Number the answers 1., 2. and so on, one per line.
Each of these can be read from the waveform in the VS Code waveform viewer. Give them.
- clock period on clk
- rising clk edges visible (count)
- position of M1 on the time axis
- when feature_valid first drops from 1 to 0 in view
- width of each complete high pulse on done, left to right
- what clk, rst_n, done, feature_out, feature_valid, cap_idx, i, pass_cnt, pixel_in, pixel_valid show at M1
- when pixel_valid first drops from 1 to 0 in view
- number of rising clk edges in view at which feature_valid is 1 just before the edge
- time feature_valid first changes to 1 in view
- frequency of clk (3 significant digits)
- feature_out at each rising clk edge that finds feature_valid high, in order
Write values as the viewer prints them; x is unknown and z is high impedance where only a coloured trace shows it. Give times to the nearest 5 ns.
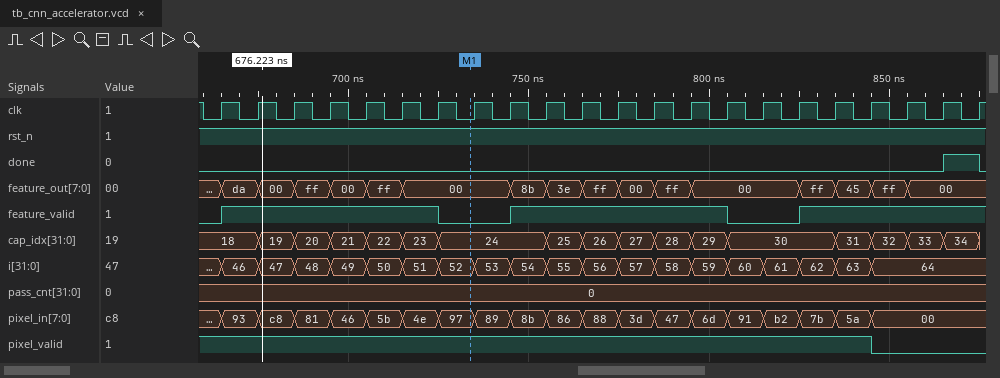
1. 10 ns
2. 22
3. 735 ns
4. 725 ns
5. 10 ns
6. clk=0, rst_n=1, done=0, feature_out=00, feature_valid=0, cap_idx=24, i=52, pass_cnt=0, pixel_in=97, pixel_valid=1
7. 845 ns
8. 17
9. 665 ns
10. 100 MHz
11. da, 00, ff, 00, ff, 00, 8b, 3e, ff, 00, ff, 00, ff, 45, ff, 00, 00
